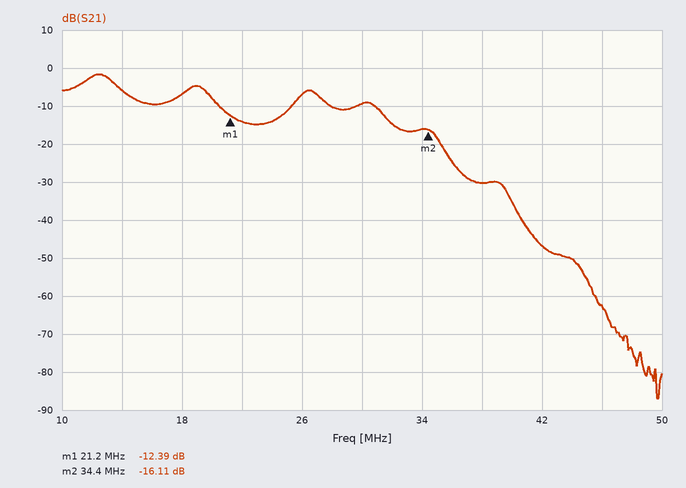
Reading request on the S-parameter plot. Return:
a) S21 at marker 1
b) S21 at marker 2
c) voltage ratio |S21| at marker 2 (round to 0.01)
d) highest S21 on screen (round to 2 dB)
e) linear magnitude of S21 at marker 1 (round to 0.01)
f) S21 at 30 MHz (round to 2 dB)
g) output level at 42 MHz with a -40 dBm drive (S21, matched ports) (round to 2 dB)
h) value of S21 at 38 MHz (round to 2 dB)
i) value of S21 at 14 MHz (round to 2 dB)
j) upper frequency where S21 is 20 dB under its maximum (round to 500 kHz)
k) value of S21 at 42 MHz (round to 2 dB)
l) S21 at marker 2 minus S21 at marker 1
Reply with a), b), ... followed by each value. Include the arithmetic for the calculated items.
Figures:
a) -12.39 dB
b) -16.11 dB
c) 10^(-16.11/20) ≈ 0.16
d) -2 dB
e) 10^(-12.39/20) ≈ 0.24
f) -10 dB
g) -40 dBm + (-46 dB) = -86 dBm
h) -30 dB
i) -6 dB
j) 35.5 MHz
k) -46 dB
l) -16.11 − (-12.39) = -3.72 dB
